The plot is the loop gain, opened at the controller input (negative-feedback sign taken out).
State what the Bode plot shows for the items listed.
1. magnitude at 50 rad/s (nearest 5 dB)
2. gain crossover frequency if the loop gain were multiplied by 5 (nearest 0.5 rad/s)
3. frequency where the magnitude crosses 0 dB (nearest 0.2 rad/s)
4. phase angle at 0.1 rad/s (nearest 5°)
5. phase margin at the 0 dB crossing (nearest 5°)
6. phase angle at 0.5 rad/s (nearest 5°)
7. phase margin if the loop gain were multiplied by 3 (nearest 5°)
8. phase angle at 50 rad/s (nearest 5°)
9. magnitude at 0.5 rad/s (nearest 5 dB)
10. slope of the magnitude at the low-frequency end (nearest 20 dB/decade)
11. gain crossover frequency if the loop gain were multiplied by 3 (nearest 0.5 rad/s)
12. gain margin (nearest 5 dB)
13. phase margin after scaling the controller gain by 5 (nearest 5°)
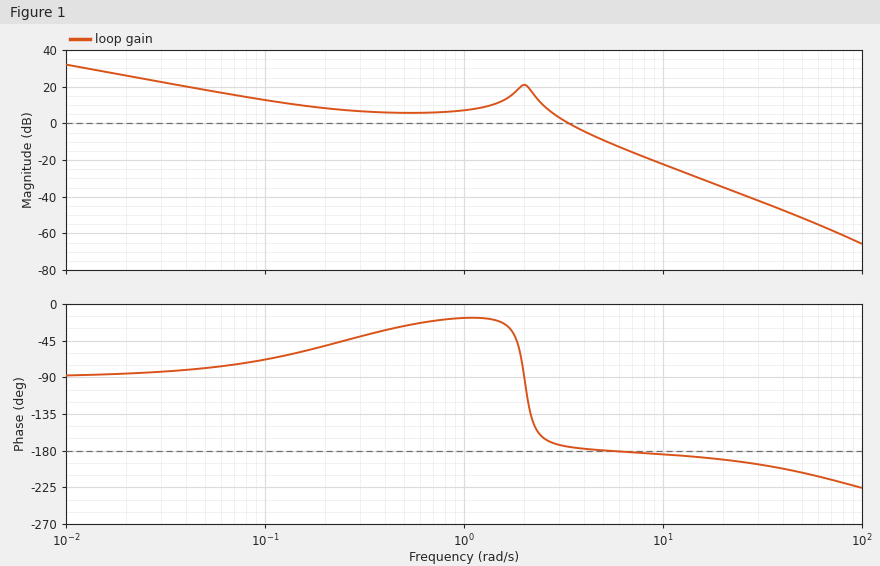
-50 dB
6.5 rad/s
3.4 rad/s
-70°
5°
-25°
0°
-205°
5 dB
-20 dB/decade
5.0 rad/s
10 dB
0°
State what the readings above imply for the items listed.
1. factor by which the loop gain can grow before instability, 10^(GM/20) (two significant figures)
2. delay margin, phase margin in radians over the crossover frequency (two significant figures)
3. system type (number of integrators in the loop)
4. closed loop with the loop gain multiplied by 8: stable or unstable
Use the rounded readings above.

3.2
0.026 s
1
unstable
